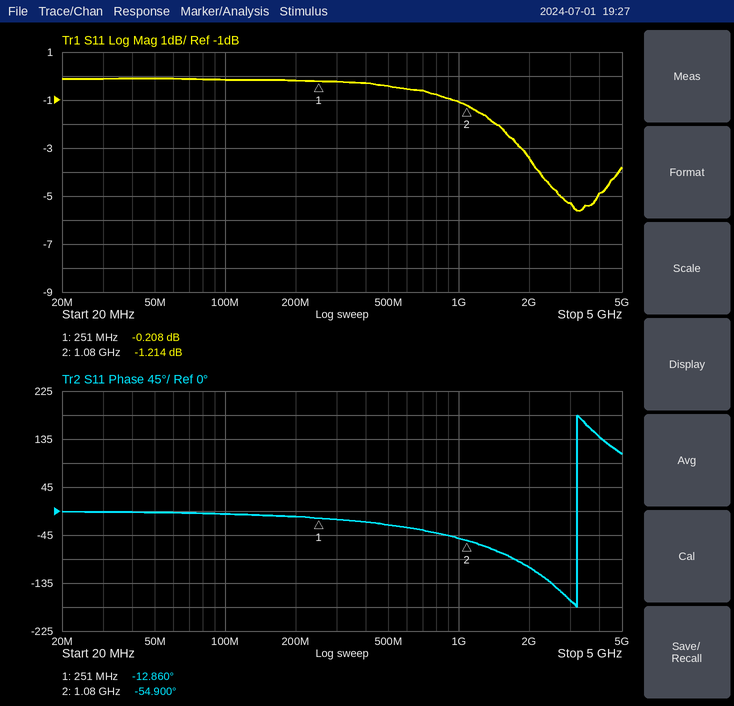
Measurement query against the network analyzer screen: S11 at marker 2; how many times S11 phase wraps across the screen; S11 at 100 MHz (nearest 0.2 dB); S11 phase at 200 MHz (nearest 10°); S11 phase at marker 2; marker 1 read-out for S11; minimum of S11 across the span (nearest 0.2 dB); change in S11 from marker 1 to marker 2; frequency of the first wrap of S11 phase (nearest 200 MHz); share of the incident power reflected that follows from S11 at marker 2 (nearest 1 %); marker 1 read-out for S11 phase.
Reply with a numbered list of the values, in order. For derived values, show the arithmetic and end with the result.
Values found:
1. -1.214 dB
2. 1
3. -0.2 dB
4. -10°
5. -54.900°
6. -0.208 dB
7. -5.6 dB
8. -1.214 − (-0.208) = -1.006 dB
9. 3.2 GHz
10. 10^(-1.214/10) ≈ 76 %
11. -12.860°
